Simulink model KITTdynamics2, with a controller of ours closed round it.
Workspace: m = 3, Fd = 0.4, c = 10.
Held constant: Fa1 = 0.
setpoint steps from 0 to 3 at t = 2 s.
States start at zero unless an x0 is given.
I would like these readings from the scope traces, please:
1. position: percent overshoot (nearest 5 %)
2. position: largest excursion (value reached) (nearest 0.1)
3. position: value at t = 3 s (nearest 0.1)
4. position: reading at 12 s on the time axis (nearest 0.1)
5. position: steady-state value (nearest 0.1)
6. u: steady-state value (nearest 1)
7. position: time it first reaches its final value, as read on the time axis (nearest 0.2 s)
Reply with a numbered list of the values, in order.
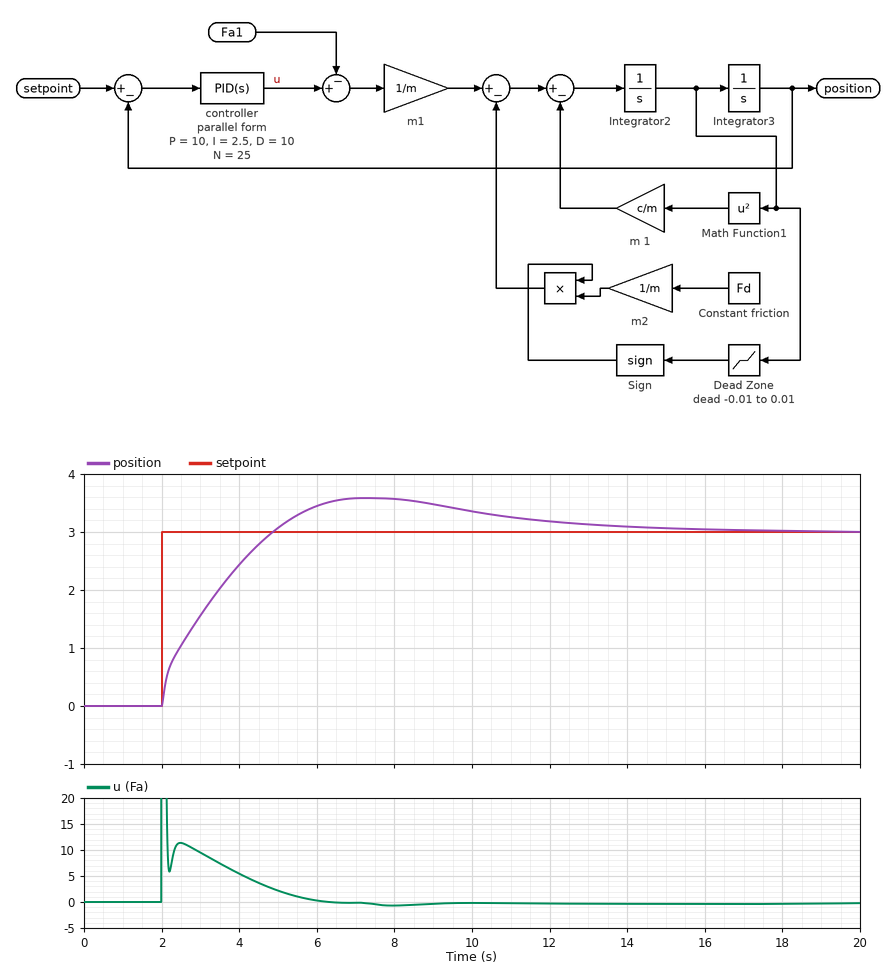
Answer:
1. 20 %
2. 3.6
3. 1.6
4. 3.2
5. 3.0
6. 0
7. 4.8 s
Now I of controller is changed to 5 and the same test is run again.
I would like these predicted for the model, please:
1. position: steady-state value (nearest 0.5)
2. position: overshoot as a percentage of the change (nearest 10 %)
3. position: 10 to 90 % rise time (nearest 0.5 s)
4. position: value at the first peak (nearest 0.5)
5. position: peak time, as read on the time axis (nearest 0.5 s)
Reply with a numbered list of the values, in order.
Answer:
1. 3.0
2. 30 %
3. 2.0 s
4. 4.0
5. 6.5 s
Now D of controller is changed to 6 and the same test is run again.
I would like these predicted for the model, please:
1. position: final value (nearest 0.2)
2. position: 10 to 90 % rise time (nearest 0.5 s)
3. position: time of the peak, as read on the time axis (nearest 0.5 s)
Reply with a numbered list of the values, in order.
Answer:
1. 3.0
2. 2.0 s
3. 6.5 s
